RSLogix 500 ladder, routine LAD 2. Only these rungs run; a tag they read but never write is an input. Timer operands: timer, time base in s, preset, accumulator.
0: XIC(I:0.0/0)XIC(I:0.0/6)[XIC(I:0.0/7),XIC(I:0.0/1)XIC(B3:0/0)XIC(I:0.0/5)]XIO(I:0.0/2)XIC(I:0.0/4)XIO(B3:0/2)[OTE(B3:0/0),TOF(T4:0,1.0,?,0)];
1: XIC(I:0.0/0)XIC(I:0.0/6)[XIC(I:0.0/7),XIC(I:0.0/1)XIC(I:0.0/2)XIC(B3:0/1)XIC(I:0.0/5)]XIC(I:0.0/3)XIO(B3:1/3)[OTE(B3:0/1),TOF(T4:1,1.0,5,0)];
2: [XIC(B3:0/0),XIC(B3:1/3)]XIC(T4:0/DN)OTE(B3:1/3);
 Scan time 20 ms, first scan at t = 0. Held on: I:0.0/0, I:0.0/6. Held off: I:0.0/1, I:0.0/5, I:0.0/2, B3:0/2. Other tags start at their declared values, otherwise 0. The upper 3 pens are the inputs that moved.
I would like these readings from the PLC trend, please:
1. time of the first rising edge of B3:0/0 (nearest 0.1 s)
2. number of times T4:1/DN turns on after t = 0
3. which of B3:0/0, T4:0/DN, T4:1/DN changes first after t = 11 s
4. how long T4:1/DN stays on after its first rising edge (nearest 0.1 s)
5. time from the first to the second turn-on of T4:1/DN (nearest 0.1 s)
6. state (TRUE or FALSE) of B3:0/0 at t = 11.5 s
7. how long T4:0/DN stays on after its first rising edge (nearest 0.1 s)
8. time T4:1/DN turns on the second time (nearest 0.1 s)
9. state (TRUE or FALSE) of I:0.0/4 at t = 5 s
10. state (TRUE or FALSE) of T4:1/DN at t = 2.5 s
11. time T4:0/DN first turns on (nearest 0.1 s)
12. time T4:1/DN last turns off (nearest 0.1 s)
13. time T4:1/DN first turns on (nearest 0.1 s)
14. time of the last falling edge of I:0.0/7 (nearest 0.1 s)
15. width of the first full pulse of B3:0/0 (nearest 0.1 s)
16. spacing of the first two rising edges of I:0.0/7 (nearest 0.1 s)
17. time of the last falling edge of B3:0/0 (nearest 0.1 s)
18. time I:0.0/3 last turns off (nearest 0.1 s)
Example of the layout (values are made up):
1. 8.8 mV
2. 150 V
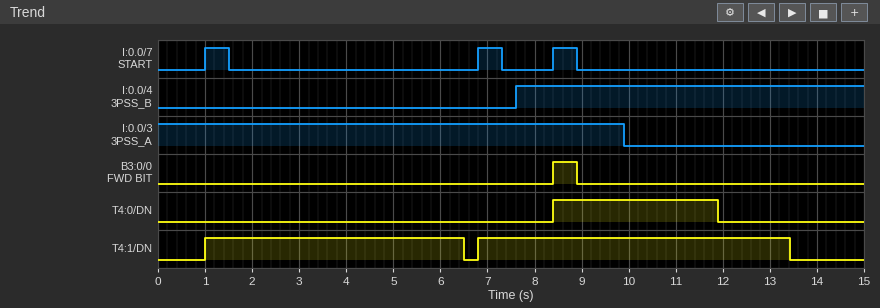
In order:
1. 8.4 s
2. 2
3. T4:0/DN
4. 5.5 s
5. 5.8 s
6. FALSE
7. 3.5 s
8. 6.8 s
9. FALSE
10. TRUE
11. 8.4 s
12. 13.4 s
13. 1.0 s
14. 8.9 s
15. 0.5 s
16. 5.8 s
17. 8.9 s
18. 9.9 s
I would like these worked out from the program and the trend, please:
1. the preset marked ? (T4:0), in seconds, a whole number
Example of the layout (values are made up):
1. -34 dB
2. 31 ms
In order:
1. 3 s
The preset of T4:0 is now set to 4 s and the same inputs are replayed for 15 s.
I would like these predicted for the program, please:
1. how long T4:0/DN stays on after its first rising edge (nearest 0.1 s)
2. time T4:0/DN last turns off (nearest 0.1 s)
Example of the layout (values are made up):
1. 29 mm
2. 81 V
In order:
1. 4.5 s
2. 12.9 s
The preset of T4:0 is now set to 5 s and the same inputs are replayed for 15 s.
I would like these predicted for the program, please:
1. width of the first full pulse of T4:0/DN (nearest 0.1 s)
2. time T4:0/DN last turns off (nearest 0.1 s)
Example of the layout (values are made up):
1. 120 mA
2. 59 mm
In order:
1. 5.5 s
2. 13.9 s
